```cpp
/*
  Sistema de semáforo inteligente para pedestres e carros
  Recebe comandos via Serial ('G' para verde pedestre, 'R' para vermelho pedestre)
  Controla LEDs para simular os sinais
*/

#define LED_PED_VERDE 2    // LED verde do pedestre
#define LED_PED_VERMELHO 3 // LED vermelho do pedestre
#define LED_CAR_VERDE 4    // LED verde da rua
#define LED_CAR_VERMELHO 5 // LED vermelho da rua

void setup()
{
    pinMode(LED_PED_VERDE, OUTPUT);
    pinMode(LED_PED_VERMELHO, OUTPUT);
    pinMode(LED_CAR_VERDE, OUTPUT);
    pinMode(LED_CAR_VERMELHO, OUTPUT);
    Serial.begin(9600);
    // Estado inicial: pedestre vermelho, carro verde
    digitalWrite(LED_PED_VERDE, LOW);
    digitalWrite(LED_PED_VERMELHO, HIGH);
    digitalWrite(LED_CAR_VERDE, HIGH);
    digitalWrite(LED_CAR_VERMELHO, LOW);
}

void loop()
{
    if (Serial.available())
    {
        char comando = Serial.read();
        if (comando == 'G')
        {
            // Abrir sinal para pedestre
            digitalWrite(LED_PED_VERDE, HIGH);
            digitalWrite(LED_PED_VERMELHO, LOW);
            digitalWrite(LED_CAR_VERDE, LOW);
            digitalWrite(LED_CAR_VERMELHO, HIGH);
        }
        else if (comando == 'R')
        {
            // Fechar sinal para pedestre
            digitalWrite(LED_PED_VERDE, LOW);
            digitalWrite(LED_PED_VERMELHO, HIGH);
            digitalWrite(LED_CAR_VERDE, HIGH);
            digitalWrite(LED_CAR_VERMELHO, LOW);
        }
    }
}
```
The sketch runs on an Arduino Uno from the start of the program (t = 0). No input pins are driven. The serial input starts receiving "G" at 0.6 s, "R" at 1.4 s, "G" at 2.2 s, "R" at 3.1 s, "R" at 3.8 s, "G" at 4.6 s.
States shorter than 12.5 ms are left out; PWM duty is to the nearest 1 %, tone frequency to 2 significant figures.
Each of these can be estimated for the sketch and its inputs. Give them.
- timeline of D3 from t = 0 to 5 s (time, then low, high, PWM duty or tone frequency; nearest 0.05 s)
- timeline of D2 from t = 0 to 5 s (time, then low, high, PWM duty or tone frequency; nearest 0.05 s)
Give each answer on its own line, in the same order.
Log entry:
0 s high; 0.6 s low; 1.4 s high; 2.2 s low; 3.1 s high; 4.6 s low
0 s low; 0.6 s high; 1.4 s low; 2.2 s high; 3.1 s low; 4.6 s high
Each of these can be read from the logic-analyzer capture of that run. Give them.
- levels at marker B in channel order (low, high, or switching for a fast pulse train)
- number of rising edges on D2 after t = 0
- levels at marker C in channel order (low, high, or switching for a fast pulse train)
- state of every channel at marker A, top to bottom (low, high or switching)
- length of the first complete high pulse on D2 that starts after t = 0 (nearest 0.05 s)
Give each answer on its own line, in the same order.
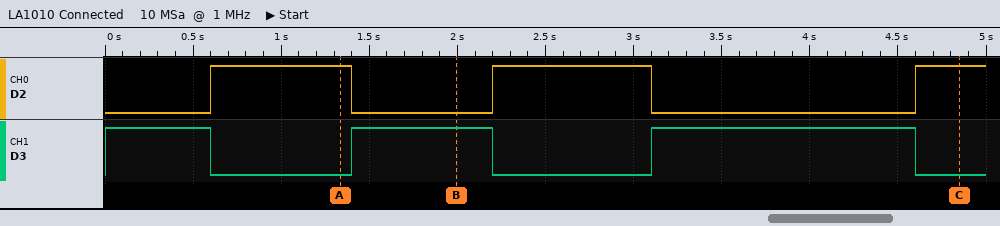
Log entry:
D2 low, D3 high
3
D2 high, D3 low
D2 high, D3 low
0.80 s
